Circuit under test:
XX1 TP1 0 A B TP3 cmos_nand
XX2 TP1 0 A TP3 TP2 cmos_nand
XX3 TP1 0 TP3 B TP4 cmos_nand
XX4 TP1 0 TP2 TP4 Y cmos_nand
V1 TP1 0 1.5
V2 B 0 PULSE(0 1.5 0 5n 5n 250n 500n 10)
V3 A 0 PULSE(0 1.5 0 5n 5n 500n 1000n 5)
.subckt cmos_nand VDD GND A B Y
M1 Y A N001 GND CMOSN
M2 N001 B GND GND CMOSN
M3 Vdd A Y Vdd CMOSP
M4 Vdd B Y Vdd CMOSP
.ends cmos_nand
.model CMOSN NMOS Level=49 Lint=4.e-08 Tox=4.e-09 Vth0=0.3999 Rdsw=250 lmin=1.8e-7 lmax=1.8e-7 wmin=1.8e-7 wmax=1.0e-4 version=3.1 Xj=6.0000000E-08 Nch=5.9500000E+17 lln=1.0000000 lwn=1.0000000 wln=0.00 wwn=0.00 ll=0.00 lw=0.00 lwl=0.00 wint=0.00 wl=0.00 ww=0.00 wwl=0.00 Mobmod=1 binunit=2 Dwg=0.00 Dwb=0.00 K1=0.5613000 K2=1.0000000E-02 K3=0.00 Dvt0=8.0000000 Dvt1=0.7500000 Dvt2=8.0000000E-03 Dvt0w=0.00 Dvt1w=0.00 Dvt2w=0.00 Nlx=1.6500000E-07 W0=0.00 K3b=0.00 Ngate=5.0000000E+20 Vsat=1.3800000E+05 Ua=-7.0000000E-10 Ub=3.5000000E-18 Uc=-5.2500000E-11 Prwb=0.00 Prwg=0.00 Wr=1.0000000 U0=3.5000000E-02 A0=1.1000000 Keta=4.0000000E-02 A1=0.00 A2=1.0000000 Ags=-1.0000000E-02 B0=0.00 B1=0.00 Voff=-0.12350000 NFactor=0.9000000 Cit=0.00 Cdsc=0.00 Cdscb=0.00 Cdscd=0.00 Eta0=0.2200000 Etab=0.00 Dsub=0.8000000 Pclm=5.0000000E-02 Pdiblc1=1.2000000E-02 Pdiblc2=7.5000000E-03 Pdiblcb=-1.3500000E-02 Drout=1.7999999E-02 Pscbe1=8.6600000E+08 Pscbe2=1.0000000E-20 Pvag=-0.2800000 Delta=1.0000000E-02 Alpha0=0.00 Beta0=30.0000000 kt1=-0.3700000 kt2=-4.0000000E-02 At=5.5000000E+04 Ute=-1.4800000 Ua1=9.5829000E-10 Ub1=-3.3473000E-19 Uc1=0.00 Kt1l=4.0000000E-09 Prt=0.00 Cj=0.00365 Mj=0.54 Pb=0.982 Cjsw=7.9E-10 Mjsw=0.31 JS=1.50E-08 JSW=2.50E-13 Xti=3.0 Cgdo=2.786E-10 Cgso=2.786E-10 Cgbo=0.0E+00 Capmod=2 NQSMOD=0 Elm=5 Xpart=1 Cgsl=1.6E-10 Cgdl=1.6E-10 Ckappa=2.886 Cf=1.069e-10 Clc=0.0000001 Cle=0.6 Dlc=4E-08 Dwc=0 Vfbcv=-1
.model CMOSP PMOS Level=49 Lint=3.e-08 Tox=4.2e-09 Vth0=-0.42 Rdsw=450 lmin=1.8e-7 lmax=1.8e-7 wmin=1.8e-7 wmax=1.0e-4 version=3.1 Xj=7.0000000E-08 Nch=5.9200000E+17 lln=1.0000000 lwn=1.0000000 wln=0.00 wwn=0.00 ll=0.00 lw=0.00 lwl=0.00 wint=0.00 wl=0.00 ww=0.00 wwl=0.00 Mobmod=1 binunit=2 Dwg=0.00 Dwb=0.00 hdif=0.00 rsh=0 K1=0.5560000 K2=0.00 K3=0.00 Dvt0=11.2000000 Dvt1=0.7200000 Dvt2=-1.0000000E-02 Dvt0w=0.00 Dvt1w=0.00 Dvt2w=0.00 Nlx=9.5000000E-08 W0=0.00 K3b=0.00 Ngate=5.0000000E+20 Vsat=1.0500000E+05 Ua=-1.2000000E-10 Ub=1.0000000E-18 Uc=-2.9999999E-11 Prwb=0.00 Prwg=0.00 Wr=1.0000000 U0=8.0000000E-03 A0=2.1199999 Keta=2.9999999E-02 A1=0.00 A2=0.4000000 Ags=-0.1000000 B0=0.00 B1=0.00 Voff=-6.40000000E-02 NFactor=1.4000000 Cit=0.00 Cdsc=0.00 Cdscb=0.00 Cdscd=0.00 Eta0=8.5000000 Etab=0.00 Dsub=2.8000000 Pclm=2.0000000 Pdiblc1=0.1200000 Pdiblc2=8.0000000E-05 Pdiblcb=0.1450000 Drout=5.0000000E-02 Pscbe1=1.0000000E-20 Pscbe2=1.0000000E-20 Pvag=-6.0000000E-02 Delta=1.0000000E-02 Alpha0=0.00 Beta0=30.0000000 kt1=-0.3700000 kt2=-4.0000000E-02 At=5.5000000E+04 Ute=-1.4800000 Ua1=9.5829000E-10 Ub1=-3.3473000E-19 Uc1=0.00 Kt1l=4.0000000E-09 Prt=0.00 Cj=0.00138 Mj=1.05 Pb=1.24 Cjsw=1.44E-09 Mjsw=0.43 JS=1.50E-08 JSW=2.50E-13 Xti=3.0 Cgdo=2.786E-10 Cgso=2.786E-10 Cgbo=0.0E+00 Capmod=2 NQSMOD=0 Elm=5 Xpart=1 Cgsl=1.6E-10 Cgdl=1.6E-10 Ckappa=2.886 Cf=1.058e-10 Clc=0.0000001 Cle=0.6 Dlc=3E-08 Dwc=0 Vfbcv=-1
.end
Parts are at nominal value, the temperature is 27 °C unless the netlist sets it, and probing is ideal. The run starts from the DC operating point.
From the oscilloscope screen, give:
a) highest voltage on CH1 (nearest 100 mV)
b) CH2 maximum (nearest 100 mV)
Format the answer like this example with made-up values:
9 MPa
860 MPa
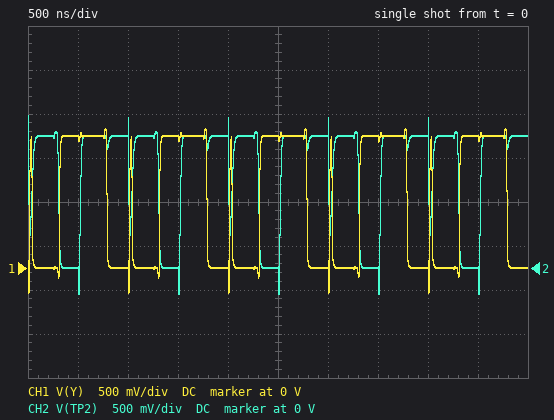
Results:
1.6 V
1.7 V
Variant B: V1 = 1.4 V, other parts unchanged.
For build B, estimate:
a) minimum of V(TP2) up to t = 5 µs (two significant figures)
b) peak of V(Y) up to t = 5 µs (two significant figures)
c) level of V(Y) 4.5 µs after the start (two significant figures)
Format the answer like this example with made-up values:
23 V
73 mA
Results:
-320 mV
1.5 V
1.4 V
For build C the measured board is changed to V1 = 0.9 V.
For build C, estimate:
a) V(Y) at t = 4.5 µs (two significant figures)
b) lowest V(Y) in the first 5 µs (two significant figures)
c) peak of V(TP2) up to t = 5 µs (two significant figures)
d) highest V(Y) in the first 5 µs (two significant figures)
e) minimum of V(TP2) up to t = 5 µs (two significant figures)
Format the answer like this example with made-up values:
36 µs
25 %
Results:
900 mV
-170 mV
1.1 V
1.0 V
-380 mV
